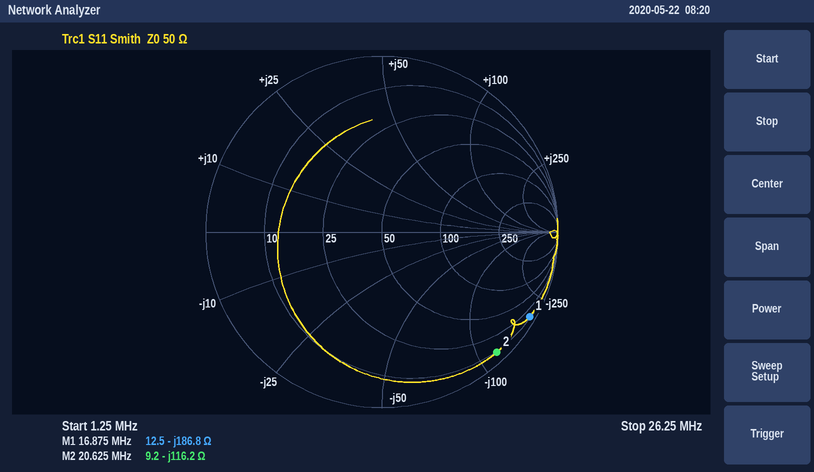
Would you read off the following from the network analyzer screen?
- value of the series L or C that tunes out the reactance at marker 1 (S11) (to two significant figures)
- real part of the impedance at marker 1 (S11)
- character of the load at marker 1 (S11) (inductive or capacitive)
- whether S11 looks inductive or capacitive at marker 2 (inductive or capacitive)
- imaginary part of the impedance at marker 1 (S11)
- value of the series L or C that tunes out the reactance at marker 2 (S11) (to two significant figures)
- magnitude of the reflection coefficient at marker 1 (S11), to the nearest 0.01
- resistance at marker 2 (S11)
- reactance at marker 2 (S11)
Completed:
1.8 µH
12.5 Ω
capacitive
capacitive
-186.8 Ω
900 nH
0.97
9.2 Ω
-116.2 Ω
